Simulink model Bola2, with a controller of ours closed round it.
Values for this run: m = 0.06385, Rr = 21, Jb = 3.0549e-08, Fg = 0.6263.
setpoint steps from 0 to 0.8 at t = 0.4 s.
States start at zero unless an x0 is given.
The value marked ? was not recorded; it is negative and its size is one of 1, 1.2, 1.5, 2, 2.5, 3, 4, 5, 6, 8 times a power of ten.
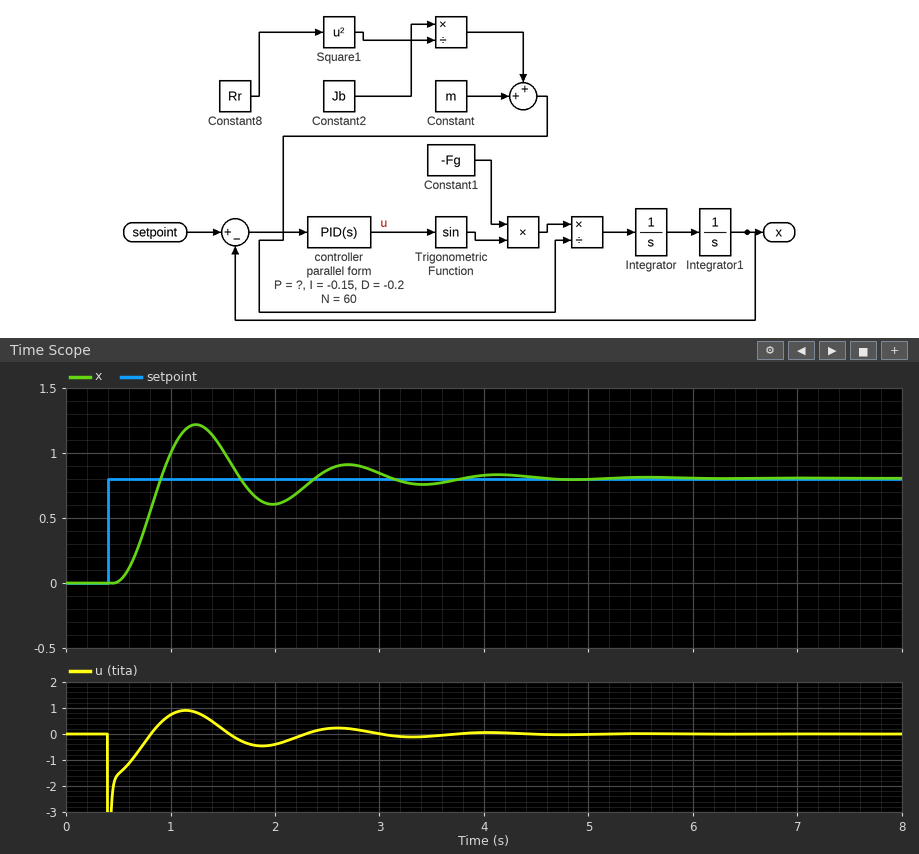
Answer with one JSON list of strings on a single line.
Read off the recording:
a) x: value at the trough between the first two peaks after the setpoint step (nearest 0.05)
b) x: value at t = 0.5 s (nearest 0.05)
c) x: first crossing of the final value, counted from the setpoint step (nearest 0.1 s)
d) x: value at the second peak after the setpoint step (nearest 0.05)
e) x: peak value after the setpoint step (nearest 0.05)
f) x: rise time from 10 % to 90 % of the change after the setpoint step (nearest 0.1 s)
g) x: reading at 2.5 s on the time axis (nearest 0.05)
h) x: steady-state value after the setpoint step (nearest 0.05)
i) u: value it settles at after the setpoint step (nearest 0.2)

["0.60", "0.00", "0.5 s", "0.90", "1.20", "0.3 s", "0.85", "0.80", "0.0"]
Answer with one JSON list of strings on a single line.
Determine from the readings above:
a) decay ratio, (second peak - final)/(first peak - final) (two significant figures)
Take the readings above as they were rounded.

["0.25"]
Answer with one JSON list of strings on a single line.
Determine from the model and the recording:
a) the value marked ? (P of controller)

["-2"]
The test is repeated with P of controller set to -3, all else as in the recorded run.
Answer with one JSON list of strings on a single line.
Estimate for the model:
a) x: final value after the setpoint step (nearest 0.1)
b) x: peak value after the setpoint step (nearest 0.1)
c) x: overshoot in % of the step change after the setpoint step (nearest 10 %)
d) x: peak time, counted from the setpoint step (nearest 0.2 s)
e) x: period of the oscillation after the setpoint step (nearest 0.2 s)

["0.8", "1.3", "60 %", "0.8 s", "1.2 s"]
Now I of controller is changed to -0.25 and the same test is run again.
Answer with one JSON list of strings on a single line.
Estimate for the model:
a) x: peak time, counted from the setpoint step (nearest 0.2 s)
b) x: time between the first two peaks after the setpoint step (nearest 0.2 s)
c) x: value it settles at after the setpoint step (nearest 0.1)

["0.8 s", "1.4 s", "0.8"]
